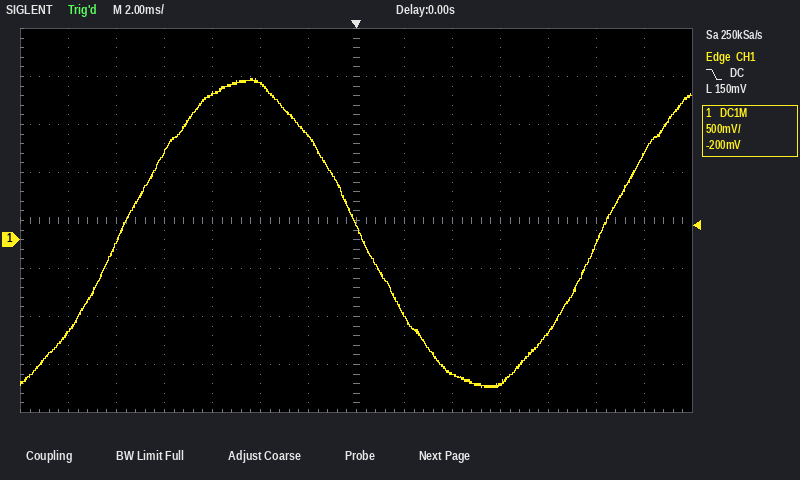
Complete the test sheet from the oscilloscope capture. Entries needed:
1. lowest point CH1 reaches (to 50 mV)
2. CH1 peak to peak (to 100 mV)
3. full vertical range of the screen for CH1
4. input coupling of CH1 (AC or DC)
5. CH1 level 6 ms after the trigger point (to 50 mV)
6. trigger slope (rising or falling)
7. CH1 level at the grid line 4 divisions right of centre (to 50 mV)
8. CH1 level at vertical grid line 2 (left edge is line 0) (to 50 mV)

-1.55 V
3.20 V
4 V
DC
-1.50 V
falling
-950 mV
-50 mV
